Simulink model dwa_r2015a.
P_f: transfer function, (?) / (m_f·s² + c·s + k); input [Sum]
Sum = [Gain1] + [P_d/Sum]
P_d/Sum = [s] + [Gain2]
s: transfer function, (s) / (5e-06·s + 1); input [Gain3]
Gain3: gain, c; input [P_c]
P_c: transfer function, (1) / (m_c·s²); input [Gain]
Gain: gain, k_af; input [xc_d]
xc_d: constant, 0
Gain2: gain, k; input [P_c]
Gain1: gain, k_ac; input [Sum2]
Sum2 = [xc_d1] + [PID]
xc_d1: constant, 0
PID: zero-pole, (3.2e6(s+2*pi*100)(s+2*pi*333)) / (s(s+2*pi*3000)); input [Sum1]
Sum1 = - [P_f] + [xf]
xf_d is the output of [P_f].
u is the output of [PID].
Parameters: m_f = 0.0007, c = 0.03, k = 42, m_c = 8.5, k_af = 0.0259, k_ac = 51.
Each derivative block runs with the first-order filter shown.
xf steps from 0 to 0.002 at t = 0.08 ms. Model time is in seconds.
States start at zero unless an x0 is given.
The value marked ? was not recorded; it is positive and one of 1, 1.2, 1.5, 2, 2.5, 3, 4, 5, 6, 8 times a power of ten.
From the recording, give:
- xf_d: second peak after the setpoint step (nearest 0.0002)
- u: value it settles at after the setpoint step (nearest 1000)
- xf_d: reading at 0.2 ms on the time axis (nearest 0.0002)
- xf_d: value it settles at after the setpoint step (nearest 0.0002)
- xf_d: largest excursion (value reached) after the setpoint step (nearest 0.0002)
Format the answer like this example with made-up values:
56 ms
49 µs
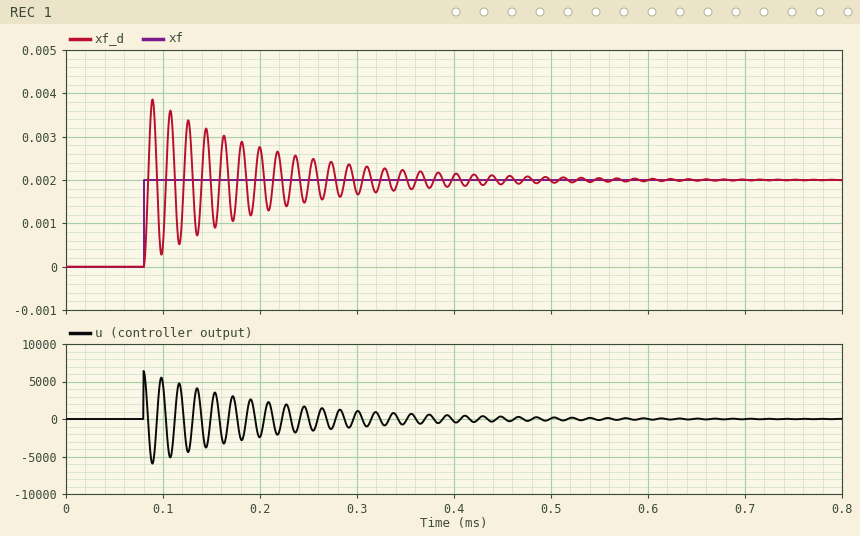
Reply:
0.0036
0
0.0028
0.0020
0.0038
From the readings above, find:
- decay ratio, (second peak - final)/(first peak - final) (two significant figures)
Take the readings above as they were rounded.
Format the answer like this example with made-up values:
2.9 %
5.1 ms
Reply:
0.89
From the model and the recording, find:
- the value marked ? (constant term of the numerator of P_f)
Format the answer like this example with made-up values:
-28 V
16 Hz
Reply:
0.5
